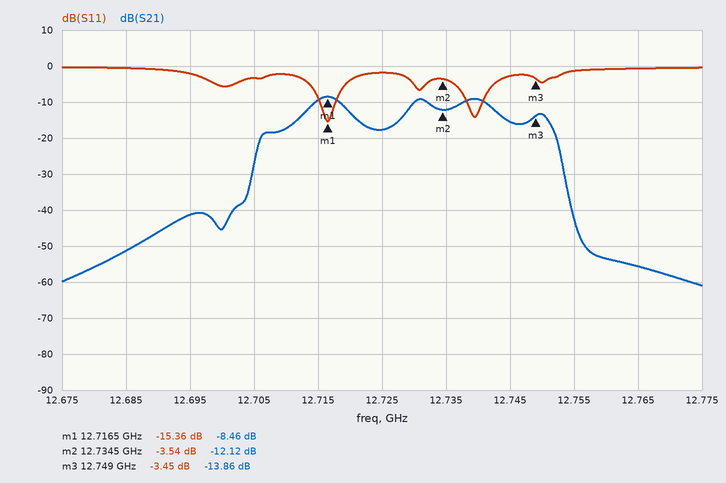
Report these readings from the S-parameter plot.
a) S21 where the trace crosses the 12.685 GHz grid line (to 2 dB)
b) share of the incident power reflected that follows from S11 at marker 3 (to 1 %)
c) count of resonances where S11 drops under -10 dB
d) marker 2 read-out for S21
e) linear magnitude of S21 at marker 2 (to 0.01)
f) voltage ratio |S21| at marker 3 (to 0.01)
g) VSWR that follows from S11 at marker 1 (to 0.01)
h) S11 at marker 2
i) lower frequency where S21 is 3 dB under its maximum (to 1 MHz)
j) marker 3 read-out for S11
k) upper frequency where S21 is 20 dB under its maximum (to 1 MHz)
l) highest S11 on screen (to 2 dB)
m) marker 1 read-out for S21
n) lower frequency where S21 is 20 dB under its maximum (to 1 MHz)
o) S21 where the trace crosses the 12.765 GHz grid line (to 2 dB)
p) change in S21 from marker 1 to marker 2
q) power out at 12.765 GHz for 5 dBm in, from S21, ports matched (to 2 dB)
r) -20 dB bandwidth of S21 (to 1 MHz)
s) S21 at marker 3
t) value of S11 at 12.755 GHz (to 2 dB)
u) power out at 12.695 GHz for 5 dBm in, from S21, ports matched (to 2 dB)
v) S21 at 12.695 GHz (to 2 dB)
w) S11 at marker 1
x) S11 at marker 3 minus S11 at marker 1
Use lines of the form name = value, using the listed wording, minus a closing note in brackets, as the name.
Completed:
S21 where the trace crosses the 12.685 GHz grid line = -52 dB
share of the incident power reflected that follows from S11 at marker 3 = 45 %
count of resonances where S11 drops under -10 dB = 2
marker 2 read-out for S21 = -12.12 dB
linear magnitude of S21 at marker 2 = 0.25
voltage ratio |S21| at marker 3 = 0.20
VSWR that follows from S11 at marker 1 = 1.41
S11 at marker 2 = -3.54 dB
lower frequency where S21 is 3 dB under its maximum = 12.714 GHz
marker 3 read-out for S11 = -3.45 dB
upper frequency where S21 is 20 dB under its maximum = 12.753 GHz
highest S11 on screen = 0 dB
marker 1 read-out for S21 = -8.46 dB
lower frequency where S21 is 20 dB under its maximum = 12.705 GHz
S21 where the trace crosses the 12.765 GHz grid line = -56 dB
change in S21 from marker 1 to marker 2 = -3.66 dB
power out at 12.765 GHz for 5 dBm in, from S21, ports matched = -50 dBm
-20 dB bandwidth of S21 = 48 MHz
S21 at marker 3 = -13.86 dB
value of S11 at 12.755 GHz = -2 dB
power out at 12.695 GHz for 5 dBm in, from S21, ports matched = -36 dBm
S21 at 12.695 GHz = -42 dB
S11 at marker 1 = -15.36 dB
S11 at marker 3 minus S11 at marker 1 = 11.91 dB
